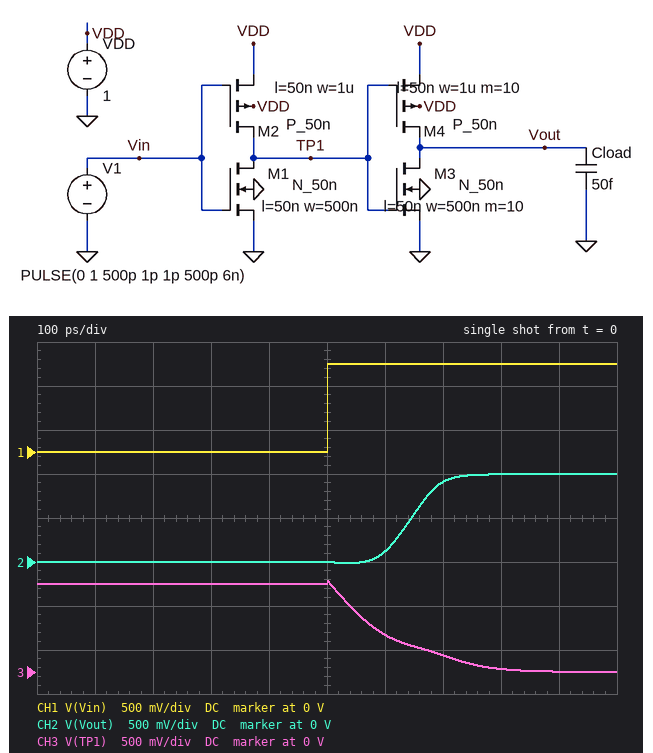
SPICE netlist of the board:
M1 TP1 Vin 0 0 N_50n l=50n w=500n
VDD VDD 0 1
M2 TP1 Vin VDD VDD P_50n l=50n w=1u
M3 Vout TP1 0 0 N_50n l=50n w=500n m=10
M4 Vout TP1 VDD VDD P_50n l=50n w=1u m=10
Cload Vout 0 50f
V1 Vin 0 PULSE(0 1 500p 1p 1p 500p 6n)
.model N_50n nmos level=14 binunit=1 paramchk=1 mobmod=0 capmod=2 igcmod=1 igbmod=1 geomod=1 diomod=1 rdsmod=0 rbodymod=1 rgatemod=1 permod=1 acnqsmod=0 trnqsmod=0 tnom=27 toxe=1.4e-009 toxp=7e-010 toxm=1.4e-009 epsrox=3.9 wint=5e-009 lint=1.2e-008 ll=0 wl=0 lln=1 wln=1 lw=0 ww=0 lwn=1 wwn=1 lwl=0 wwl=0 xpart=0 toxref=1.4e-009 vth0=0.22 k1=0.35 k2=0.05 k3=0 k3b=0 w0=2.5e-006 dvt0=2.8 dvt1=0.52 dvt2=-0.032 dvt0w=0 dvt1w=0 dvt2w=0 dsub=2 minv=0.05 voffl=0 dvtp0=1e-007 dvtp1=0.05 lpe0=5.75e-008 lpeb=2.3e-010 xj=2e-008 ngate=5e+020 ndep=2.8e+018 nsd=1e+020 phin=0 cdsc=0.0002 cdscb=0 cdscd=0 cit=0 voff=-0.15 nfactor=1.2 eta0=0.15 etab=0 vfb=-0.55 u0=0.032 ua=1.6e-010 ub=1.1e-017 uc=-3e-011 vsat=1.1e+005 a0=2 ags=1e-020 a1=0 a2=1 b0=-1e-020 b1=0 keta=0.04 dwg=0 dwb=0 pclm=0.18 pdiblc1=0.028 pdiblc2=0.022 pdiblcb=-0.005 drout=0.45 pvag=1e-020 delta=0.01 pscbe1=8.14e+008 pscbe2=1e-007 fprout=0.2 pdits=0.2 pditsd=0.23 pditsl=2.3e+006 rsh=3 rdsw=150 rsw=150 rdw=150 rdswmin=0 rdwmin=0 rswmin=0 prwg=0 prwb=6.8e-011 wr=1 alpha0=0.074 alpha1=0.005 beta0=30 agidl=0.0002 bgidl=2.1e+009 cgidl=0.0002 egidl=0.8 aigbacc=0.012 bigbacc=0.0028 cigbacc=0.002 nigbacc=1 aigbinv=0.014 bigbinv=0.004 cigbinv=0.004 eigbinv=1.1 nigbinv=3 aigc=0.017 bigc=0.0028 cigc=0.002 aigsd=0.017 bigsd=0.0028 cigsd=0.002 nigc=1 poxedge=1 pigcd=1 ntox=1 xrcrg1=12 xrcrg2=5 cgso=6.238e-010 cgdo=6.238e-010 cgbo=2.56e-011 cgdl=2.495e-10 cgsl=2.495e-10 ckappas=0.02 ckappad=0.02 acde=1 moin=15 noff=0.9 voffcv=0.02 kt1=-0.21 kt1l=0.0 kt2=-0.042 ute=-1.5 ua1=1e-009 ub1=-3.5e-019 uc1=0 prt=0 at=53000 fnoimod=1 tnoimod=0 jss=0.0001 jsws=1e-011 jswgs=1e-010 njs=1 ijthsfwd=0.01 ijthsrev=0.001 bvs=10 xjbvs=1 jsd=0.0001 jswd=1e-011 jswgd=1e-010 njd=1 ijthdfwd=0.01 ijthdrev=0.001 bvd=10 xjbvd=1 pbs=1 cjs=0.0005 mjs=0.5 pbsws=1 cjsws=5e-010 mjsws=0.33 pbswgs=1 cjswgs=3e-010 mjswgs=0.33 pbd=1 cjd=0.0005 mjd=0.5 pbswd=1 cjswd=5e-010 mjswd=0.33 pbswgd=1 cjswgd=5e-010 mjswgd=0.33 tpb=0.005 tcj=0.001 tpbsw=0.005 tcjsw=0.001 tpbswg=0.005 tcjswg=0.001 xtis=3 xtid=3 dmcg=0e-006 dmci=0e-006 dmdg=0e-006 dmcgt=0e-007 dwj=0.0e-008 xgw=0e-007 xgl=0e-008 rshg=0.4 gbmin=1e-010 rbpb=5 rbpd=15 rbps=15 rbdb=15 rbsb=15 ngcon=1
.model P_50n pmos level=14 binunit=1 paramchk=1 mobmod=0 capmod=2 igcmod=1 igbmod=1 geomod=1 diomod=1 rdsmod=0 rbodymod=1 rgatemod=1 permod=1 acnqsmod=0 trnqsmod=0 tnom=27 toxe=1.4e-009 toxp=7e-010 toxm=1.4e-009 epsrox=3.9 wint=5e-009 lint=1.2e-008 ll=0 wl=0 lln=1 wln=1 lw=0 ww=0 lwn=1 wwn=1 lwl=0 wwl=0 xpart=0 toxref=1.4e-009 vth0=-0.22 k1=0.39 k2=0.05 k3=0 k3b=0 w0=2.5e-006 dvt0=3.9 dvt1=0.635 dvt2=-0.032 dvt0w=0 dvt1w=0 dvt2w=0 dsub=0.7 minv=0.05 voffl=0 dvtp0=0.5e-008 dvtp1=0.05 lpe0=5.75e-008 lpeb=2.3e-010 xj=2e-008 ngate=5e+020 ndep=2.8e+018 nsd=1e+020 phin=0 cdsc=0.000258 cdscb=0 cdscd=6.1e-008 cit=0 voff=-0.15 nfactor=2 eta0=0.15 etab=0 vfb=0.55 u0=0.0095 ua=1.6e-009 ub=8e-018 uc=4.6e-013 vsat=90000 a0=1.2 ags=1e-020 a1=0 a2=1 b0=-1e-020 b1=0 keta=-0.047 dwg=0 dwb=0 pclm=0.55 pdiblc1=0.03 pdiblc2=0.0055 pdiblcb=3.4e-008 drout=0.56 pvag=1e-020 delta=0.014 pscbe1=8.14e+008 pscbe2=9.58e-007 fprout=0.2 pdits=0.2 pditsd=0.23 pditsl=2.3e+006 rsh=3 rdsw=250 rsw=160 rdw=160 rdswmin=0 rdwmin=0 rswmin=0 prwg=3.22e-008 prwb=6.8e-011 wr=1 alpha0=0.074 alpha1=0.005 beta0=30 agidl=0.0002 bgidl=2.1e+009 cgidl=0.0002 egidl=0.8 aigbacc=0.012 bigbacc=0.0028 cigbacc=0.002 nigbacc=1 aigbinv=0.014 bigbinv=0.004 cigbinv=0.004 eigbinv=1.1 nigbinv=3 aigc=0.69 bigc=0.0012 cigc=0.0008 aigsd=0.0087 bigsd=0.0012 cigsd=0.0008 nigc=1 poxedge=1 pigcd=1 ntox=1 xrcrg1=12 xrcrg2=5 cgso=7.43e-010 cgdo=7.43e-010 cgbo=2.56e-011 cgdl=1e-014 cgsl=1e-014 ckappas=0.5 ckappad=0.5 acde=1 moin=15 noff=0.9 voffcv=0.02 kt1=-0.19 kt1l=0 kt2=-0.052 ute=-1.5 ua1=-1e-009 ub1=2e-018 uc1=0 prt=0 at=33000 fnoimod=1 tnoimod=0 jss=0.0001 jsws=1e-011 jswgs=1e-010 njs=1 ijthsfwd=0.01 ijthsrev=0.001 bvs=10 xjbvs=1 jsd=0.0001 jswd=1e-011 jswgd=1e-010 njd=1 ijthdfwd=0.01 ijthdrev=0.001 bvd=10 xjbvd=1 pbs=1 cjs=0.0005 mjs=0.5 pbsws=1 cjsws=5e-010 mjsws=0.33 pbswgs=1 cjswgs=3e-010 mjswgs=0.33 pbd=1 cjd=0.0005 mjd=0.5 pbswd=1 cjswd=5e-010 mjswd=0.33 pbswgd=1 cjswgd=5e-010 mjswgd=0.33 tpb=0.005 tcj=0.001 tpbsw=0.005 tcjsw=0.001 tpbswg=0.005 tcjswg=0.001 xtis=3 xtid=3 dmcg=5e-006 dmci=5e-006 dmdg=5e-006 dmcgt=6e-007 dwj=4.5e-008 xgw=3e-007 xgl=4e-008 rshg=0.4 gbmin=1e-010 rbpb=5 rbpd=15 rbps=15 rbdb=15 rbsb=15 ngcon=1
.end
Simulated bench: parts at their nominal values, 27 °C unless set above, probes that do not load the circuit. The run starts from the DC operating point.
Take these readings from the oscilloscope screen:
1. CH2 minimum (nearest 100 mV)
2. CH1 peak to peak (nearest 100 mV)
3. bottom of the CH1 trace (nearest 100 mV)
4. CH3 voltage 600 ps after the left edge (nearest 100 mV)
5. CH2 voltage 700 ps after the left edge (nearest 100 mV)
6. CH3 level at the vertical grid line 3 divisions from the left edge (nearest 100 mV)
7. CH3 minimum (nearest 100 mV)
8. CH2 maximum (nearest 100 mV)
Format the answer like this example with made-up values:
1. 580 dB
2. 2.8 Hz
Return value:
1. 0 V
2. 1.0 V
3. 0 V
4. 400 mV
5. 900 mV
6. 1.0 V
7. 0 V
8. 1.0 V
